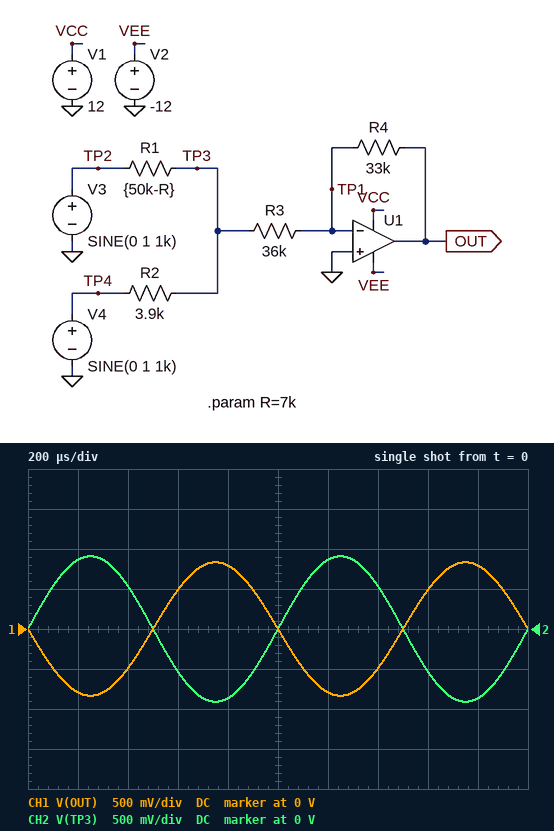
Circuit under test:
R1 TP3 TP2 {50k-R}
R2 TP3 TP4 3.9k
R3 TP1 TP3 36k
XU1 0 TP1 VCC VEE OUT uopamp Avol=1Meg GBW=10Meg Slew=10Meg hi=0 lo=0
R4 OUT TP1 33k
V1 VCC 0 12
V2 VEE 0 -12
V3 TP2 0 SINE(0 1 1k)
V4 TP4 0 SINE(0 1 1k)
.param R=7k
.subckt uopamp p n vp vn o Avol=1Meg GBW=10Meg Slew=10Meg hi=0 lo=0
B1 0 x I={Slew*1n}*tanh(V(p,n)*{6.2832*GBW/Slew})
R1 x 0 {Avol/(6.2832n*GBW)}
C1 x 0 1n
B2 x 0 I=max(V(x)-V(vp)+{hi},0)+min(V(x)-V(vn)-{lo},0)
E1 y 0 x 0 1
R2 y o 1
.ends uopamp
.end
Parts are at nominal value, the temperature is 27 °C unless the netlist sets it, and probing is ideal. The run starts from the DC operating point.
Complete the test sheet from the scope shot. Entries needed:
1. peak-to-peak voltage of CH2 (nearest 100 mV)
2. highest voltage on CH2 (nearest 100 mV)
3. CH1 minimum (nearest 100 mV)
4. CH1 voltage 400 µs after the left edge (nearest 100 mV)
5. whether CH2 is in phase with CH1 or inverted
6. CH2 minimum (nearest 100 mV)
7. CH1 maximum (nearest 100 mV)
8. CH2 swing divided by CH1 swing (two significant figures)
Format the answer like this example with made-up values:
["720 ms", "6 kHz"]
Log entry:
["1.8 V", "900 mV", "-800 mV", "-500 mV", "inverted", "-900 mV", "800 mV", "1.1"]
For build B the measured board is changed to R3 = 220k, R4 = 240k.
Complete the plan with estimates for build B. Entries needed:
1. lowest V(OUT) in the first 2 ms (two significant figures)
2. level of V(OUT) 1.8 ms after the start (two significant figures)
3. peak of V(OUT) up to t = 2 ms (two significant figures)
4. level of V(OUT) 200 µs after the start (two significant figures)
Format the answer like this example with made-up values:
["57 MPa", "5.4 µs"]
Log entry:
["-1.1 V", "1.0 V", "1.1 V", "-1.0 V"]
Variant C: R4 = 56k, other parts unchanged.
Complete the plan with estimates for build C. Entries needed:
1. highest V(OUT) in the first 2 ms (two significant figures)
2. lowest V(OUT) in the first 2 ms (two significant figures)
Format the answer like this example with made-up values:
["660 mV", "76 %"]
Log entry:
["1.4 V", "-1.4 V"]
